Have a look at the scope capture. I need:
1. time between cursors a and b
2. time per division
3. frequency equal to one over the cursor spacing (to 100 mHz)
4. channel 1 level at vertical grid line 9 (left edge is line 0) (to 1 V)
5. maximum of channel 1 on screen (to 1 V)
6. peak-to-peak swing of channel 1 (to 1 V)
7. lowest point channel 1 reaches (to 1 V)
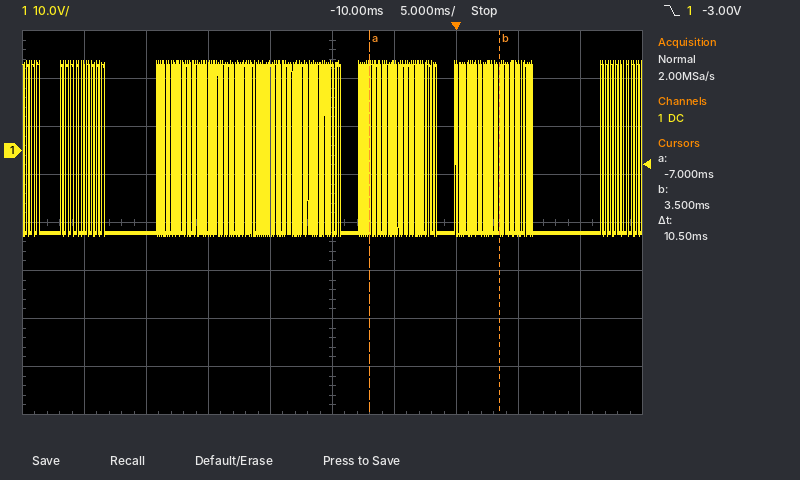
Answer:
10.5 ms
5 ms
95.2 Hz
-17 V
19 V
37 V
-18 V
